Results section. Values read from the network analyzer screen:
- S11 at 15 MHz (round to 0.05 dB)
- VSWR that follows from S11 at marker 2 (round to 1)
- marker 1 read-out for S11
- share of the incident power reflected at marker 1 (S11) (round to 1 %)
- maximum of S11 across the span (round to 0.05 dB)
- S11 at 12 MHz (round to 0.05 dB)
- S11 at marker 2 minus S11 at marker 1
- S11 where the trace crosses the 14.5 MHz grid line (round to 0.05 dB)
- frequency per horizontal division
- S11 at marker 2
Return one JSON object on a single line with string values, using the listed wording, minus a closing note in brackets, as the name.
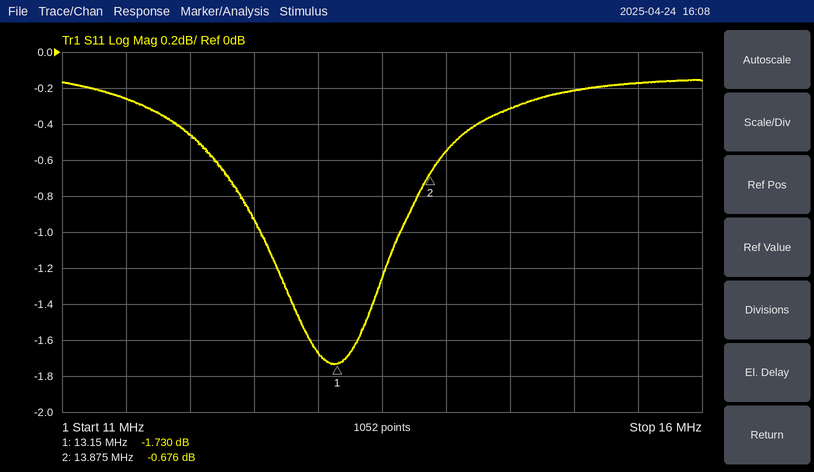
{"S11 at 15 MHz": "-0.20 dB", "VSWR that follows from S11 at marker 2": "26", "marker 1 read-out for S11": "-1.730 dB", "share of the incident power reflected at marker 1 (S11)": "67 %", "maximum of S11 across the span": "-0.15 dB", "S11 at 12 MHz": "-0.45 dB", "S11 at marker 2 minus S11 at marker 1": "1.054 dB", "S11 where the trace crosses the 14.5 MHz grid line": "-0.30 dB", "frequency per horizontal division": "500 kHz", "S11 at marker 2": "-0.676 dB"}
